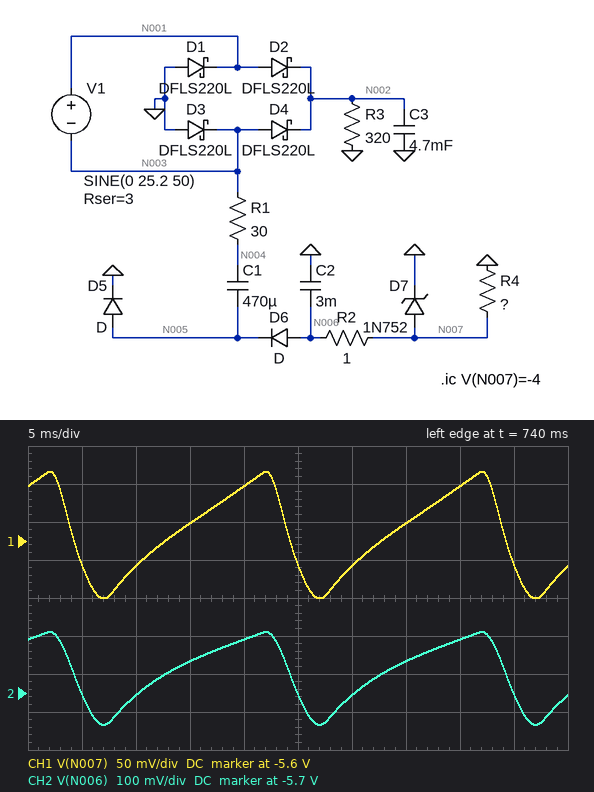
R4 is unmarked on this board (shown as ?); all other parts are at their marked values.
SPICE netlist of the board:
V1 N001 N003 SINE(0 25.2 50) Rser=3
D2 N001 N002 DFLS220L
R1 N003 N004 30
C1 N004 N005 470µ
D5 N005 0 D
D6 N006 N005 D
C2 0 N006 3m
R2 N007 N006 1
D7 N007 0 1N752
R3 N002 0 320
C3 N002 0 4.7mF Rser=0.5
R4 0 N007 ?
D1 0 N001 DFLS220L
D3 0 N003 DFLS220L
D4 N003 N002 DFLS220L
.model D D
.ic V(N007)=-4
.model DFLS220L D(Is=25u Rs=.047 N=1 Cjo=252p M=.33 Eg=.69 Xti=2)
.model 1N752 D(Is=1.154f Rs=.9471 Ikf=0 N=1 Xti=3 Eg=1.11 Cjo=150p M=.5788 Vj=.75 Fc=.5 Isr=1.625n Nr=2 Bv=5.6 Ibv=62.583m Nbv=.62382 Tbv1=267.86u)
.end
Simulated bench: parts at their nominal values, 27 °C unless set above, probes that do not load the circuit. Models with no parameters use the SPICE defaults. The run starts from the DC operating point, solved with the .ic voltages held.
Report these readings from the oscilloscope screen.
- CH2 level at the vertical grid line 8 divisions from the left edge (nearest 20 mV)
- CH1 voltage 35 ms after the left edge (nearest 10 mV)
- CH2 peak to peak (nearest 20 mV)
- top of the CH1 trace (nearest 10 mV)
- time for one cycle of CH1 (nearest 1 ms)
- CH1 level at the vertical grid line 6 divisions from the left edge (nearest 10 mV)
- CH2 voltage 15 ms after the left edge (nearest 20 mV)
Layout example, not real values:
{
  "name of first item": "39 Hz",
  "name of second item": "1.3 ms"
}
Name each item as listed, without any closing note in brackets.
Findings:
{
  "CH2 level at the vertical grid line 8 divisions from the left edge": "-5.56 V",
  "CH1 voltage 35 ms after the left edge": "-5.58 V",
  "CH2 peak to peak": "240 mV",
  "top of the CH1 trace": "-5.51 V",
  "time for one cycle of CH1": "20 ms",
  "CH1 level at the vertical grid line 6 divisions from the left edge": "-5.63 V",
  "CH2 voltage 15 ms after the left edge": "-5.62 V"
}
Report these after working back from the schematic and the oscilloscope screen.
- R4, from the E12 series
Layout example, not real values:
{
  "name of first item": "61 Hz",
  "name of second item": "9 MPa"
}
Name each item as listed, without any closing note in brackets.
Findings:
{
  "R4, from the E12 series": "180 Ω"
}
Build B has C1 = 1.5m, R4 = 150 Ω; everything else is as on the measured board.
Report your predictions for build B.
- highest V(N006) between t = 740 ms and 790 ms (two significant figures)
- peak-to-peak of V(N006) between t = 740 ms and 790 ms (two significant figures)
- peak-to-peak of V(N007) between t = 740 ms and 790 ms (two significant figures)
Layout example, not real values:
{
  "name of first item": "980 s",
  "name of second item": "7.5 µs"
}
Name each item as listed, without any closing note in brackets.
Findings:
{
  "highest V(N006) between t = 740 ms and 790 ms": "-5.5 V",
  "peak-to-peak of V(N006) between t = 740 ms and 790 ms": "250 mV",
  "peak-to-peak of V(N007) between t = 740 ms and 790 ms": "180 mV"
}
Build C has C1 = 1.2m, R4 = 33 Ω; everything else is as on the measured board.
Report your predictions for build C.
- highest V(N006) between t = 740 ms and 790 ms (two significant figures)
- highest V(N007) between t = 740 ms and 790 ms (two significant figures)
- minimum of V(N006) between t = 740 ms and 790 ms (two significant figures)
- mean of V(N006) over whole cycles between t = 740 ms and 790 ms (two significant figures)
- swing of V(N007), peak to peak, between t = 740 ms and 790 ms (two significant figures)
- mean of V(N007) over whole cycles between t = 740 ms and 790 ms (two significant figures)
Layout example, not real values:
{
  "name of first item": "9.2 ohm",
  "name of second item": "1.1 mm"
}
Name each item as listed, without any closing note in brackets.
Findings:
{
  "highest V(N006) between t = 740 ms and 790 ms": "-2.2 V",
  "highest V(N007) between t = 740 ms and 790 ms": "-2.1 V",
  "minimum of V(N006) between t = 740 ms and 790 ms": "-2.5 V",
  "mean of V(N006) over whole cycles between t = 740 ms and 790 ms": "-2.4 V",
  "swing of V(N007), peak to peak, between t = 740 ms and 790 ms": "320 mV",
  "mean of V(N007) over whole cycles between t = 740 ms and 790 ms": "-2.3 V"
}
